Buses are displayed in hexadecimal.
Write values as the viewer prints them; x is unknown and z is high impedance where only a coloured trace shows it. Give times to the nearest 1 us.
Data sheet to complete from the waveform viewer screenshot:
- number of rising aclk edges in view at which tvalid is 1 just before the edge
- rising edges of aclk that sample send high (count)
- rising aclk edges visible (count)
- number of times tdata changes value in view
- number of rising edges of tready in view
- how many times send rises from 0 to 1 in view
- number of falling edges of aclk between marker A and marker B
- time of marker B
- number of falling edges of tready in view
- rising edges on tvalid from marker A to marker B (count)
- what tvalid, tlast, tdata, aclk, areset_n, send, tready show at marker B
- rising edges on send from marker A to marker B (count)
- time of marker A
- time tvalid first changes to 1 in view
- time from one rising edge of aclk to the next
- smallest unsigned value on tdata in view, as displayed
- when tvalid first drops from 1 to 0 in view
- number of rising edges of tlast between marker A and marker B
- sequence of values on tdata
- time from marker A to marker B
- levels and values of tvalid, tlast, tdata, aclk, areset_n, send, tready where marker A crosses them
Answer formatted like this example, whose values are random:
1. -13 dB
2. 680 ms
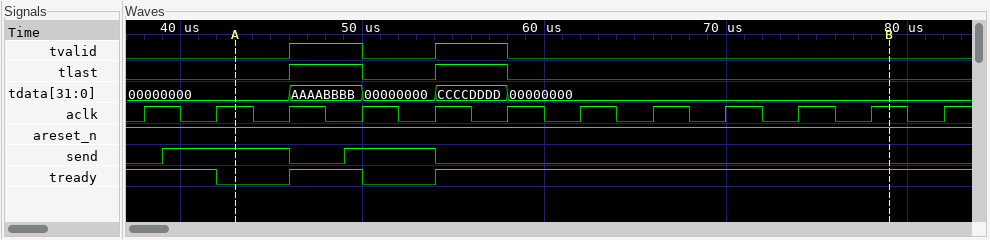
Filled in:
1. 2
2. 4
3. 12
4. 4
5. 2
6. 2
7. 9
8. 79 us
9. 2
10. 2
11. tvalid=0, tlast=0, tdata=00000000, aclk=1, areset_n=1, send=0, tready=1
12. 1
13. 43 us
14. 46 us
15. 4 us
16. 00000000
17. 50 us
18. 2
19. 00000000, AAAABBBB, 00000000, CCCCDDDD, 00000000
20. 36 us
21. tvalid=0, tlast=0, tdata=00000000, aclk=1, areset_n=1, send=1, tready=0
